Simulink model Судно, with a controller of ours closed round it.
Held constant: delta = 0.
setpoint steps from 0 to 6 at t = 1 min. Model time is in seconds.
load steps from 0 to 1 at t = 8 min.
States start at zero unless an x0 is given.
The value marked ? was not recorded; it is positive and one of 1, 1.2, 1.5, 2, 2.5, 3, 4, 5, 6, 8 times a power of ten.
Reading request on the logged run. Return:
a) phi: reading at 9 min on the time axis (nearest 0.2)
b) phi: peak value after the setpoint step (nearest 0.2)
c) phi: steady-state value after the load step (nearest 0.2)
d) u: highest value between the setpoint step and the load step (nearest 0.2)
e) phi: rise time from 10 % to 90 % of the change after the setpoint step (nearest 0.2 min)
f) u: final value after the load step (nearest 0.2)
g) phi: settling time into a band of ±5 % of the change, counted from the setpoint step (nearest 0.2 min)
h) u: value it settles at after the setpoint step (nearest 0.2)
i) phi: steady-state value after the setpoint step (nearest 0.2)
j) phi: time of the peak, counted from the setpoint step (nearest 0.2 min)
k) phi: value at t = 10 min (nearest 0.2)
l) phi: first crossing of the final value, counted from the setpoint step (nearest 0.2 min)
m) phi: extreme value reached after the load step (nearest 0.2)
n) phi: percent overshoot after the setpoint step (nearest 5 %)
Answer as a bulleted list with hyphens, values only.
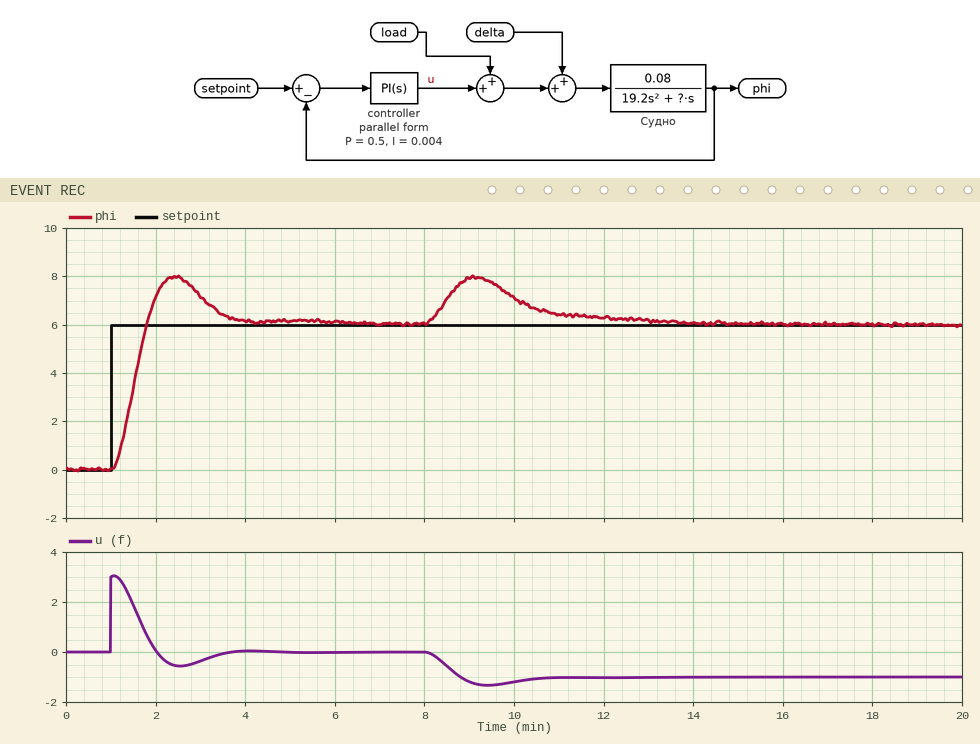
- 8.0
- 8.0
- 6.0
- 3.0
- 0.6 min
- -1.0
- 2.6 min
- 0.0
- 6.0
- 1.4 min
- 7.2
- 0.8 min
- 8.0
- 35 %
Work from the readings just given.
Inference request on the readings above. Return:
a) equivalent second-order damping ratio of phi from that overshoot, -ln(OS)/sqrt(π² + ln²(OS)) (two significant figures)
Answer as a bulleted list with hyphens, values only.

- 0.32
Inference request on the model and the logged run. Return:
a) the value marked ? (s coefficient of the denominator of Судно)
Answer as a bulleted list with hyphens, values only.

- 1
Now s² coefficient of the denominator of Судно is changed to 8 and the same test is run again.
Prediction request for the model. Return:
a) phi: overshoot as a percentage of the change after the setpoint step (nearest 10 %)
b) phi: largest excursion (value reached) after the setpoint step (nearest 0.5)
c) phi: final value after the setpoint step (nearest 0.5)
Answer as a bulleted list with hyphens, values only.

- 20 %
- 7.0
- 6.0
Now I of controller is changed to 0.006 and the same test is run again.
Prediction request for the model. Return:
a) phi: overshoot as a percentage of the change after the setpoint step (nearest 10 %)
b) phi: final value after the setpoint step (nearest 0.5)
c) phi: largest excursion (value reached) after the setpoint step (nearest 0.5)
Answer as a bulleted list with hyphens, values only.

- 40 %
- 6.0
- 8.5
